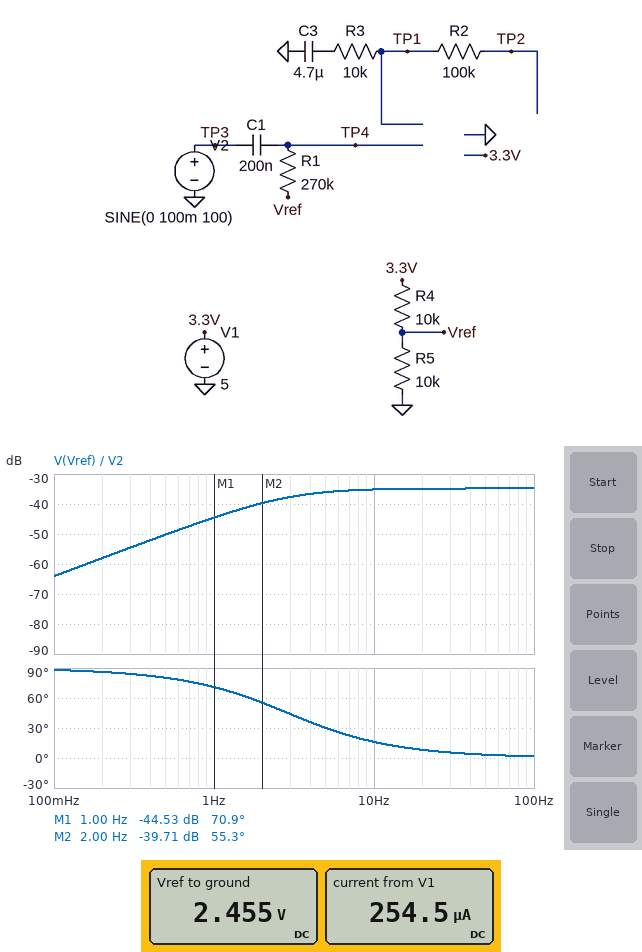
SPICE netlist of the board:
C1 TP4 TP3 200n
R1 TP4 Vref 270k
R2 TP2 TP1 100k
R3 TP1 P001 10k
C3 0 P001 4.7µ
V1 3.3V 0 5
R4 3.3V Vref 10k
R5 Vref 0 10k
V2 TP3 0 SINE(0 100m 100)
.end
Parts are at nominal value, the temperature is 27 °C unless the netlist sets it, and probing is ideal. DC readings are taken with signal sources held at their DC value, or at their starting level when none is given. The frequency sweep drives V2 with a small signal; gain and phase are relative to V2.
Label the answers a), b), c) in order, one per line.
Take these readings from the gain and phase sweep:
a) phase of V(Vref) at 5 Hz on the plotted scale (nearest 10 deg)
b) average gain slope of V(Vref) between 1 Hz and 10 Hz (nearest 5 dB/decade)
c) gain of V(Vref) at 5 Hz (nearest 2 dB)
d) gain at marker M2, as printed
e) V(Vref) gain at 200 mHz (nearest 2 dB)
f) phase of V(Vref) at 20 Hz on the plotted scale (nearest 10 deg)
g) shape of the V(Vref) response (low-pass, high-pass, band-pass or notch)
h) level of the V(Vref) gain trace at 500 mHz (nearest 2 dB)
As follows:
a) 30 deg
b) 10 dB/decade
c) -36 dB
d) -39.71 dB
e) -58 dB
f) 10 deg
g) high-pass
h) -50 dB
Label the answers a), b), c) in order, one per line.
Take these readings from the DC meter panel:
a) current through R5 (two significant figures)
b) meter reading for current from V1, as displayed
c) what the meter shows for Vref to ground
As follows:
a) 250 µA
b) 254.5 µA
c) 2.455 V
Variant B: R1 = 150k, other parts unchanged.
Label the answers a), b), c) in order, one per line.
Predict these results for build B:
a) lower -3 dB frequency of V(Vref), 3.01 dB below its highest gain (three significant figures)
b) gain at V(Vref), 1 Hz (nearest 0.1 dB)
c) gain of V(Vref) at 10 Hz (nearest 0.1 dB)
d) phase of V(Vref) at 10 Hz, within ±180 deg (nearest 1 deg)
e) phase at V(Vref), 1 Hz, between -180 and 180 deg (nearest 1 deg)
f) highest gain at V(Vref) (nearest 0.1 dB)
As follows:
a) 5.13 Hz
b) -44.2 dB
c) -30.8 dB
d) 27 deg
e) 79 deg
f) -29.8 dB
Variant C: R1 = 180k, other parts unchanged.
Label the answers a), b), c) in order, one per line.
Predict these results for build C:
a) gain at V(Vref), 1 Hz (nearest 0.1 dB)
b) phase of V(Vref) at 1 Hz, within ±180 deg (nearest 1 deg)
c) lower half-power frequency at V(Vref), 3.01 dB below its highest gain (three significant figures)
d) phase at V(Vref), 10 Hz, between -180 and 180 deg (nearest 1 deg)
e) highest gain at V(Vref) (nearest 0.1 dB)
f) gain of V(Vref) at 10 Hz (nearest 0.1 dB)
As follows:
a) -44.3 dB
b) 77 deg
c) 4.30 Hz
d) 23 deg
e) -31.4 dB
f) -32.1 dB
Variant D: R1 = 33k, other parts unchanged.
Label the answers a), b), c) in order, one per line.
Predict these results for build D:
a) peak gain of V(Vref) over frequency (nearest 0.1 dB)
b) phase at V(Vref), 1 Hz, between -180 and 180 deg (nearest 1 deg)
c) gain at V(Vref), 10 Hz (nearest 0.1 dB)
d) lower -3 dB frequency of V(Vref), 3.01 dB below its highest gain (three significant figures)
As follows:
a) -17.6 dB
b) 87 deg
c) -24.9 dB
d) 20.9 Hz
